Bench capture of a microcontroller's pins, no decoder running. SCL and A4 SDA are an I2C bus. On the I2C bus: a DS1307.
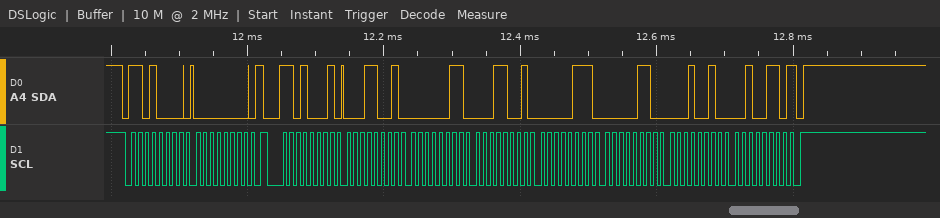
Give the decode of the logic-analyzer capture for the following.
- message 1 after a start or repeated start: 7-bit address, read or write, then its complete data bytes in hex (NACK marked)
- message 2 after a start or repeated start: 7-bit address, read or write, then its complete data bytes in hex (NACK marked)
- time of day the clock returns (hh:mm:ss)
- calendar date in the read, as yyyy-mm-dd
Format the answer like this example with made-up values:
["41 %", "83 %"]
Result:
["0x68 write: 00", "0x68 read: 19 03 19 07 06 12 26 NACK", "19:03:19", "2026-12-06"]
